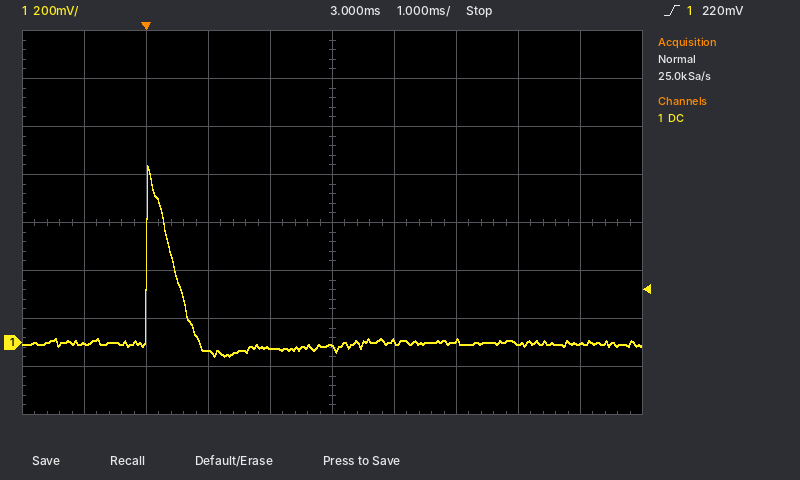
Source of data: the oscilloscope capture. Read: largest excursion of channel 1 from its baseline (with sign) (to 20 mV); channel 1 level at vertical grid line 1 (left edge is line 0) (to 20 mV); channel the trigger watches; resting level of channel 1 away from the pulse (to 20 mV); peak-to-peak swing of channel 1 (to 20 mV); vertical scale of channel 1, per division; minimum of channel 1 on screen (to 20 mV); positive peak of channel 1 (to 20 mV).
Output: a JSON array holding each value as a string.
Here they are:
["+740 mV", "0 mV", "channel 1", "0 mV", "800 mV", "200 mV", "-60 mV", "740 mV"]
